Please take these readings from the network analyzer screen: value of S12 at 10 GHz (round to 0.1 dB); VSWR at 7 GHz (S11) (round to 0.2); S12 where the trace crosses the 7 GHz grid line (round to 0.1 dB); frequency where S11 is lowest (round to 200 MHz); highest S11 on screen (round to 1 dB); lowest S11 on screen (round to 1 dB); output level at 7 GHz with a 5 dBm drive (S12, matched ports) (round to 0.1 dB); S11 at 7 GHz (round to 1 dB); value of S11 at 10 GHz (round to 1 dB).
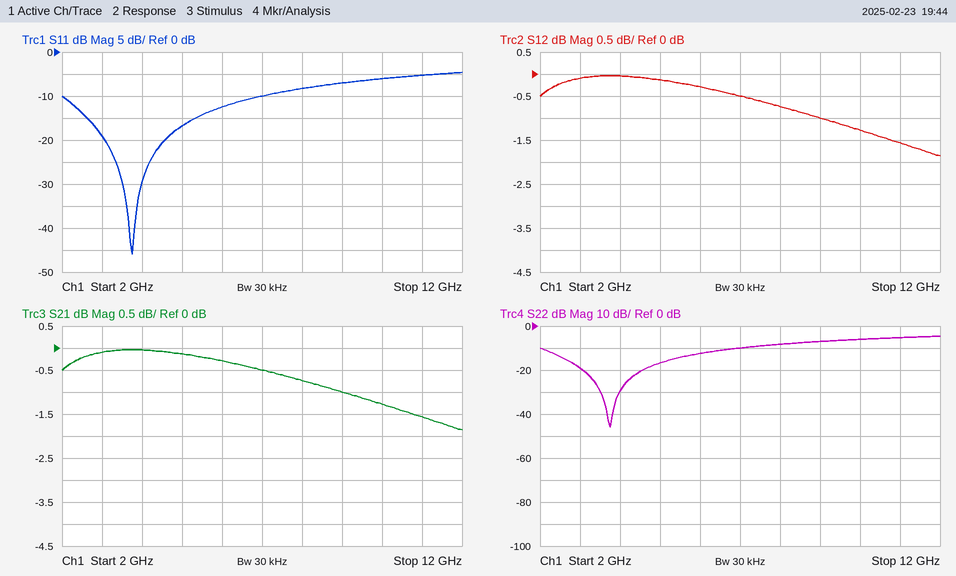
-1.3 dB
2.0
-0.5 dB
3.8 GHz
-5 dB
-46 dB
4.5 dBm
-10 dB
-6 dB
